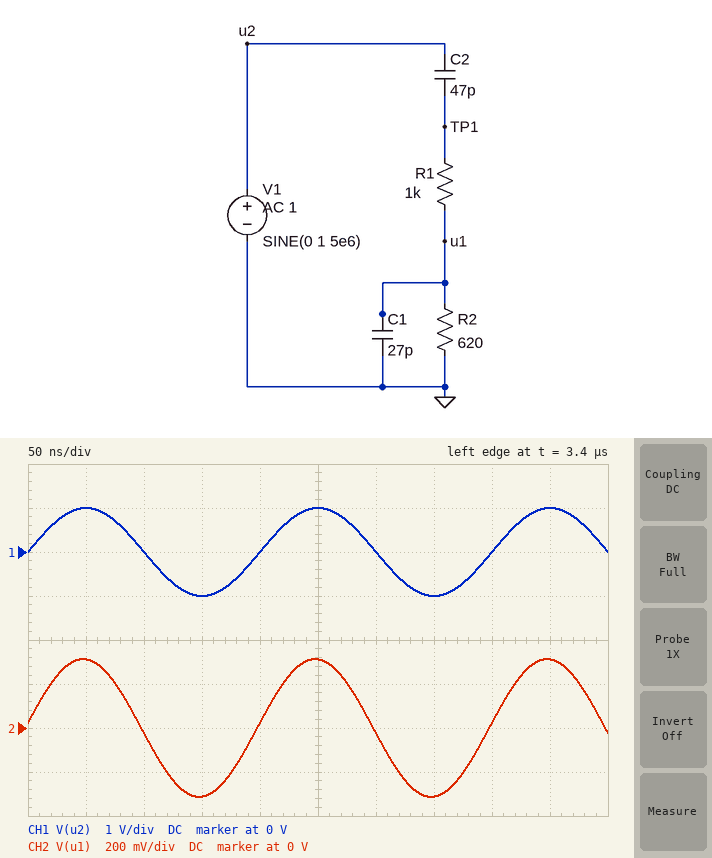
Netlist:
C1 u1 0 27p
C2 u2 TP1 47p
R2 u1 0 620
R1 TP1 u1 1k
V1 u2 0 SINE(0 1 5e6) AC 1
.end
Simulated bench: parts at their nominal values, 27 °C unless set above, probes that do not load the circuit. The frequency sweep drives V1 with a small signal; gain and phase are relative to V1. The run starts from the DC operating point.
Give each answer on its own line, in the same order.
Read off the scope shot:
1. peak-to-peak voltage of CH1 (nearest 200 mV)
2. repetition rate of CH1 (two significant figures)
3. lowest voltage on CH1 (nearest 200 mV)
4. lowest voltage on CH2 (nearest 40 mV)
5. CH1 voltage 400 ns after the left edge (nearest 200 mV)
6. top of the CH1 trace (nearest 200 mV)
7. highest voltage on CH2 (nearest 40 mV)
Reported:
2.0 V
5.0 MHz
-1.0 V
-320 mV
0 V
1.0 V
320 mV
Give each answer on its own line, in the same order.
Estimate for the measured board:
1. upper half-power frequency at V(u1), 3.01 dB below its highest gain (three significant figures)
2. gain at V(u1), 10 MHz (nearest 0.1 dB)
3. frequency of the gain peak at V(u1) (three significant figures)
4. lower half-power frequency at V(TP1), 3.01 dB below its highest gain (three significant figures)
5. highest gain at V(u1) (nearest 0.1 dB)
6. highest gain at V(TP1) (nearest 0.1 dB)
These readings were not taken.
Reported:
20.4 MHz
-10.6 dB
5.67 MHz
2.33 MHz
-10.1 dB
0 dB
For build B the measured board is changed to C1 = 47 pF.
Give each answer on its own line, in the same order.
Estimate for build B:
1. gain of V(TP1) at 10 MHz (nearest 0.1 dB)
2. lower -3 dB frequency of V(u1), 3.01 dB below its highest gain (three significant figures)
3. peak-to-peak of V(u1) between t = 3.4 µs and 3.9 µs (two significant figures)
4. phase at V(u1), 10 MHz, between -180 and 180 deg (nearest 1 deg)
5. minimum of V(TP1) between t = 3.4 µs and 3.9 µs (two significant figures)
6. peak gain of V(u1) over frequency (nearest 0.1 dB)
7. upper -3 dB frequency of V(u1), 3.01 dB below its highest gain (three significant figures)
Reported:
-0.8 dB
1.36 MHz
550 mV
-34 deg
-830 mV
-11.2 dB
13.6 MHz
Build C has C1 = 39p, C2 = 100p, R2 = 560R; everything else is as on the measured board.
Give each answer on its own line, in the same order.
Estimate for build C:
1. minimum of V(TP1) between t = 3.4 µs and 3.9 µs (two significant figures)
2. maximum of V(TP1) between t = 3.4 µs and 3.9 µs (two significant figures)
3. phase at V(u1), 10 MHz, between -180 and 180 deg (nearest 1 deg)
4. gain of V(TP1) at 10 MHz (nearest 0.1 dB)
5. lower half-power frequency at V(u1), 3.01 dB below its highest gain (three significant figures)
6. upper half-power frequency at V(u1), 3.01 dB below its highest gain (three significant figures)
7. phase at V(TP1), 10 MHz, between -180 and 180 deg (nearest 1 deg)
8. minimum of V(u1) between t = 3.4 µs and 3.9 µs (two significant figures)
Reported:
-940 mV
940 mV
-34 deg
-0.3 dB
840 kHz
13.8 MHz
7 deg
-310 mV
